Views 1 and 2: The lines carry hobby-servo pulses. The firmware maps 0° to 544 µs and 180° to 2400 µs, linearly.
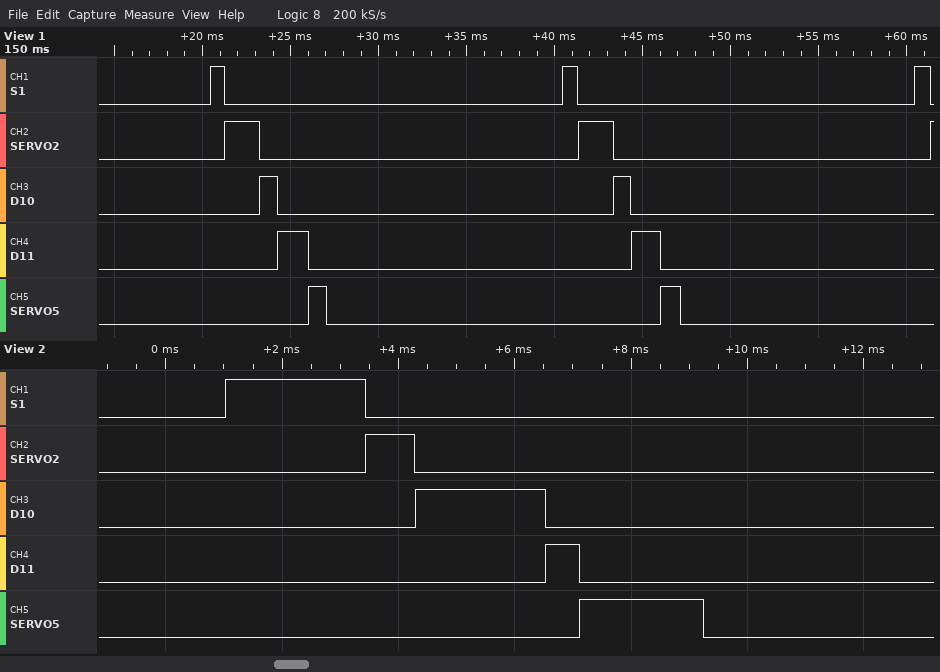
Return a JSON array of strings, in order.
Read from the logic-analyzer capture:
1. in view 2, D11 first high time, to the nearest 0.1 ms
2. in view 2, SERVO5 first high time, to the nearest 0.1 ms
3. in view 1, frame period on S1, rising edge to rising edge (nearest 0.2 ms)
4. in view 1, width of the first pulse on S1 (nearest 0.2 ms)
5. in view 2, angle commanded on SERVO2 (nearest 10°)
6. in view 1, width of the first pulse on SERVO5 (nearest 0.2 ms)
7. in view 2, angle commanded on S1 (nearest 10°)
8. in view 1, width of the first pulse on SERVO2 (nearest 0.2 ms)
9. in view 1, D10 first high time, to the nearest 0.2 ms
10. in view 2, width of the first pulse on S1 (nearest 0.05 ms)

["0.6 ms", "2.1 ms", "20.0 ms", "0.8 ms", "30°", "1.0 ms", "180°", "2.0 ms", "1.0 ms", "2.40 ms"]
